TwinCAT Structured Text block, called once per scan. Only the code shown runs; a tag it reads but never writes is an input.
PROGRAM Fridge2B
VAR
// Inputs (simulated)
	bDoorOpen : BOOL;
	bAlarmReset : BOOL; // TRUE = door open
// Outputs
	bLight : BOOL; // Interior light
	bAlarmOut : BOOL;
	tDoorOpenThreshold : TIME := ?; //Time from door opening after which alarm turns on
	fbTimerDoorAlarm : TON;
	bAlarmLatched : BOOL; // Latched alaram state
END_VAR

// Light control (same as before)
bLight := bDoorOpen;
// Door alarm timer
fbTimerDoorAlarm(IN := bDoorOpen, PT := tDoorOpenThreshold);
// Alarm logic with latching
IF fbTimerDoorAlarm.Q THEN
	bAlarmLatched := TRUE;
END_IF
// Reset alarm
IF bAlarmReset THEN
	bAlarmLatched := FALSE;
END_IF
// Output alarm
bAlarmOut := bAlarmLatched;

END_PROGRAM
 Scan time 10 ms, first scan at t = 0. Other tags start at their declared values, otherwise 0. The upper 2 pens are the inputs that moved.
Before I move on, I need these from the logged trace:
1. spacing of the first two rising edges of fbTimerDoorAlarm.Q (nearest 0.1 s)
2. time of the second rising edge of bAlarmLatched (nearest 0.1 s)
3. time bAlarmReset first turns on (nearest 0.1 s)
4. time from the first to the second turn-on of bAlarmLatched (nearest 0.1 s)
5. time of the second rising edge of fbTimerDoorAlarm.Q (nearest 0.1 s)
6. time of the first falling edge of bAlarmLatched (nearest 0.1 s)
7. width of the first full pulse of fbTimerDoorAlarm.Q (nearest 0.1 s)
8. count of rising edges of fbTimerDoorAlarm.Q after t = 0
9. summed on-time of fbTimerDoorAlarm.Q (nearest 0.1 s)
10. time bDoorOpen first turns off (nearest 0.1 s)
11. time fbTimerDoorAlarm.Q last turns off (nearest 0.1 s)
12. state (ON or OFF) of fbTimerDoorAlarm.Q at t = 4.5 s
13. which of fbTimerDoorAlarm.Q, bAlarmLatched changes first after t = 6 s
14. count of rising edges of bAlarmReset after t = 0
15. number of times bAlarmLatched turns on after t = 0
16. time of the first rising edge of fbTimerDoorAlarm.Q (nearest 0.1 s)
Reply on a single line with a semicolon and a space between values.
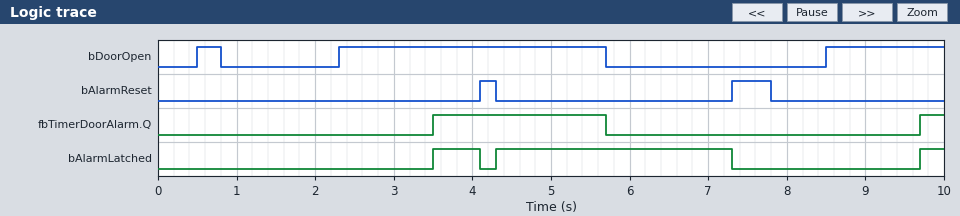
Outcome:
6.2 s; 4.3 s; 4.1 s; 0.8 s; 9.7 s; 4.1 s; 2.2 s; 2; 2.5 s; 0.8 s; 5.7 s; ON; bAlarmLatched; 2; 3; 3.5 s
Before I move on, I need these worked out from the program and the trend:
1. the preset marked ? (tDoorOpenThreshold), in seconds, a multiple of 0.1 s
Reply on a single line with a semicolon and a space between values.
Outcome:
1.2 s
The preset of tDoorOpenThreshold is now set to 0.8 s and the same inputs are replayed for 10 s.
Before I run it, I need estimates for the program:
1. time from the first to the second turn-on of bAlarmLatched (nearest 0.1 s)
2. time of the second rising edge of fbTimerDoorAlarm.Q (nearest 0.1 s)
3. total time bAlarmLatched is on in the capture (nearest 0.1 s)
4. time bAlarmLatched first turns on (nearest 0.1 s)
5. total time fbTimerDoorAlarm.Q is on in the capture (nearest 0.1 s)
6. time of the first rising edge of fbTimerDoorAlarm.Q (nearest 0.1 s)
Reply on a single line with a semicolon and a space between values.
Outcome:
1.2 s; 9.3 s; 4.7 s; 3.1 s; 3.3 s; 3.1 s
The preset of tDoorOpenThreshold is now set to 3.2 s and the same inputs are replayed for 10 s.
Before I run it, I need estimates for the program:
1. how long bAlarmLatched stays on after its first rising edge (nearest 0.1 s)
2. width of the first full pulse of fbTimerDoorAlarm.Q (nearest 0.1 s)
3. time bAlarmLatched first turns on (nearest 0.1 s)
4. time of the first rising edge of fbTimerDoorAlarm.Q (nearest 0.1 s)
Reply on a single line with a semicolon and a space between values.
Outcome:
1.8 s; 0.2 s; 5.5 s; 5.5 s
